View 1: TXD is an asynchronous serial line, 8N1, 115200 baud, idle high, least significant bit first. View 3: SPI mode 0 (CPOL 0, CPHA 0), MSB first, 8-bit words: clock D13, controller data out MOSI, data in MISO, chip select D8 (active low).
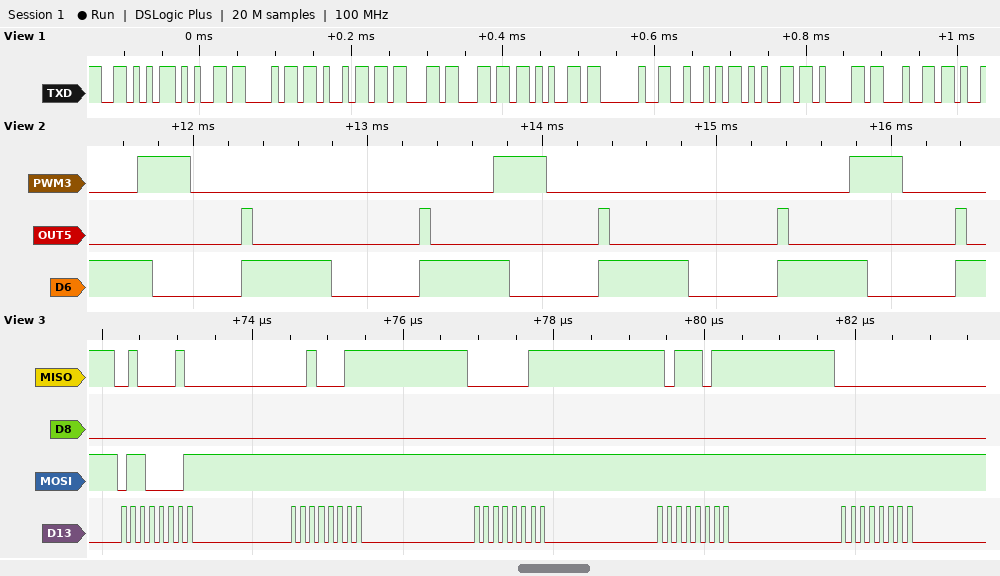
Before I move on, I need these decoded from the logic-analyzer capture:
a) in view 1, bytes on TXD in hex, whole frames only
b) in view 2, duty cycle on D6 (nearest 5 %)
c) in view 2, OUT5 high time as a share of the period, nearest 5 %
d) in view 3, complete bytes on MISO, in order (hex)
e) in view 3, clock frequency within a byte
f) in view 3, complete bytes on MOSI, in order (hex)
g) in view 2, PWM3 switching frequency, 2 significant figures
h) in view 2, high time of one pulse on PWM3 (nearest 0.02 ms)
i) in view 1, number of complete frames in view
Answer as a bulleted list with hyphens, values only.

- 56 65 68 69 63 6C 65 20 52 65 61 64
- 50 %
- 5 %
- 42 23 03 BB 00
- 8 MHz
- 61 FF FF FF FF
- 490 Hz
- 0.30 ms
- 12
